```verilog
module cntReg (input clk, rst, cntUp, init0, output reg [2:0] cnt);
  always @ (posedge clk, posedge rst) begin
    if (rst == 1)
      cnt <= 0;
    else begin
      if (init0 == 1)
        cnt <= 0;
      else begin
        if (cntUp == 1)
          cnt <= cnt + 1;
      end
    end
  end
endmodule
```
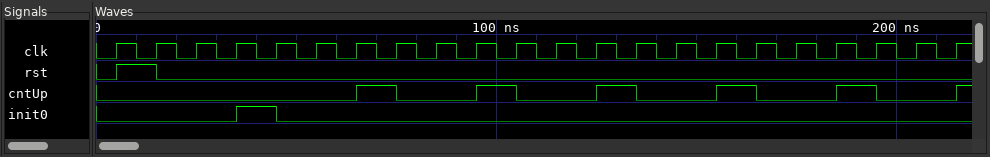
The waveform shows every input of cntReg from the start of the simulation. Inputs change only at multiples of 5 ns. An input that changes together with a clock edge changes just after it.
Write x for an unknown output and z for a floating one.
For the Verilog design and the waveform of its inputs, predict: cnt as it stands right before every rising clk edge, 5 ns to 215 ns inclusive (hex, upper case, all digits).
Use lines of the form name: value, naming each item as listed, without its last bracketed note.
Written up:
cnt as it stands right before every rising clk edge, 5 ns to 215 ns inclusive: x, 0, 0, 0, 0, 0, 0, 0, 1, 1, 1, 2, 2, 2, 3, 3, 3, 4, 4, 4, 5, 5
